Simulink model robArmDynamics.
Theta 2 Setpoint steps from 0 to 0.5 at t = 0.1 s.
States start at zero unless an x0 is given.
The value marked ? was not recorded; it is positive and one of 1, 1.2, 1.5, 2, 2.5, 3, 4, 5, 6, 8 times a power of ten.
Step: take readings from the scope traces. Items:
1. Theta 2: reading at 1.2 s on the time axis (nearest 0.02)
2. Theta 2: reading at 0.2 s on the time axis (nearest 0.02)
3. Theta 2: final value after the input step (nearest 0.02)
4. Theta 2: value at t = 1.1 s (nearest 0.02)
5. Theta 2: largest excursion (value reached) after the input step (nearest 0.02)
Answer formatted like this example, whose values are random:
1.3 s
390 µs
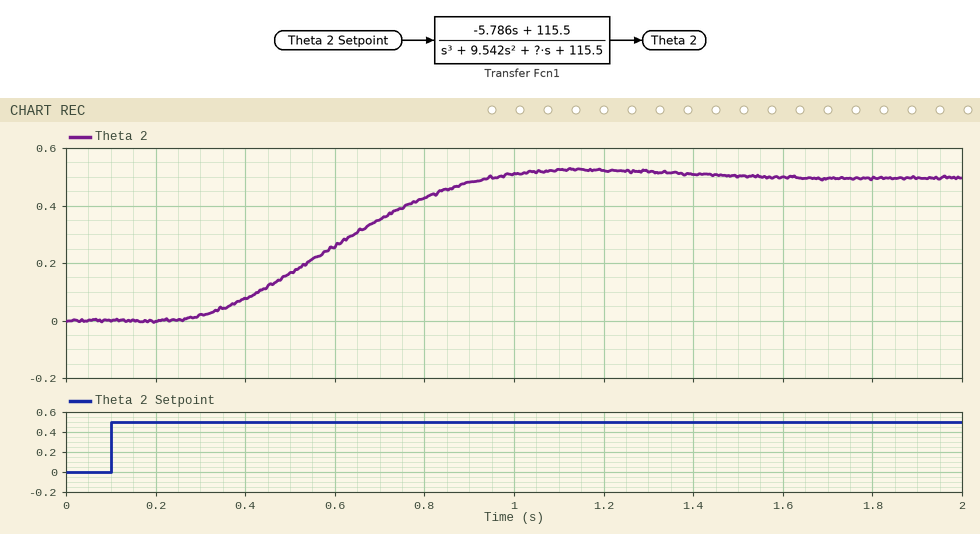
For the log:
0.52
0.00
0.50
0.52
0.52
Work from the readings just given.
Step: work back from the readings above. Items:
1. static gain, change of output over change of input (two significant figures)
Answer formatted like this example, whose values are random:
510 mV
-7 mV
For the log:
1.0
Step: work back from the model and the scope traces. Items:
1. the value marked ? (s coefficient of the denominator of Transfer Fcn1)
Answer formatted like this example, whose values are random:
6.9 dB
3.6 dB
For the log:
50
